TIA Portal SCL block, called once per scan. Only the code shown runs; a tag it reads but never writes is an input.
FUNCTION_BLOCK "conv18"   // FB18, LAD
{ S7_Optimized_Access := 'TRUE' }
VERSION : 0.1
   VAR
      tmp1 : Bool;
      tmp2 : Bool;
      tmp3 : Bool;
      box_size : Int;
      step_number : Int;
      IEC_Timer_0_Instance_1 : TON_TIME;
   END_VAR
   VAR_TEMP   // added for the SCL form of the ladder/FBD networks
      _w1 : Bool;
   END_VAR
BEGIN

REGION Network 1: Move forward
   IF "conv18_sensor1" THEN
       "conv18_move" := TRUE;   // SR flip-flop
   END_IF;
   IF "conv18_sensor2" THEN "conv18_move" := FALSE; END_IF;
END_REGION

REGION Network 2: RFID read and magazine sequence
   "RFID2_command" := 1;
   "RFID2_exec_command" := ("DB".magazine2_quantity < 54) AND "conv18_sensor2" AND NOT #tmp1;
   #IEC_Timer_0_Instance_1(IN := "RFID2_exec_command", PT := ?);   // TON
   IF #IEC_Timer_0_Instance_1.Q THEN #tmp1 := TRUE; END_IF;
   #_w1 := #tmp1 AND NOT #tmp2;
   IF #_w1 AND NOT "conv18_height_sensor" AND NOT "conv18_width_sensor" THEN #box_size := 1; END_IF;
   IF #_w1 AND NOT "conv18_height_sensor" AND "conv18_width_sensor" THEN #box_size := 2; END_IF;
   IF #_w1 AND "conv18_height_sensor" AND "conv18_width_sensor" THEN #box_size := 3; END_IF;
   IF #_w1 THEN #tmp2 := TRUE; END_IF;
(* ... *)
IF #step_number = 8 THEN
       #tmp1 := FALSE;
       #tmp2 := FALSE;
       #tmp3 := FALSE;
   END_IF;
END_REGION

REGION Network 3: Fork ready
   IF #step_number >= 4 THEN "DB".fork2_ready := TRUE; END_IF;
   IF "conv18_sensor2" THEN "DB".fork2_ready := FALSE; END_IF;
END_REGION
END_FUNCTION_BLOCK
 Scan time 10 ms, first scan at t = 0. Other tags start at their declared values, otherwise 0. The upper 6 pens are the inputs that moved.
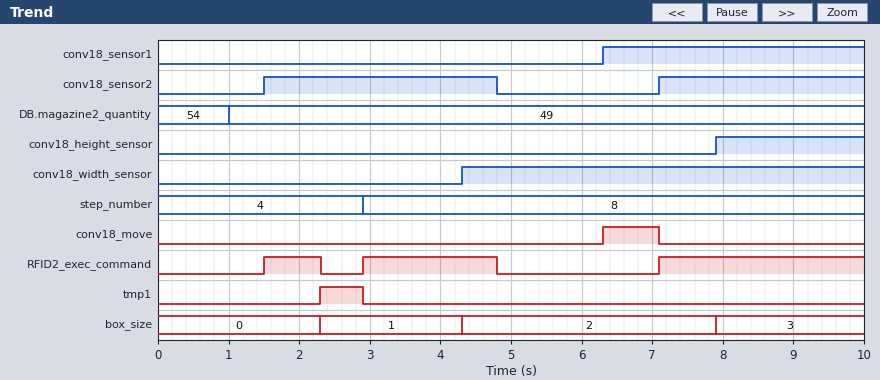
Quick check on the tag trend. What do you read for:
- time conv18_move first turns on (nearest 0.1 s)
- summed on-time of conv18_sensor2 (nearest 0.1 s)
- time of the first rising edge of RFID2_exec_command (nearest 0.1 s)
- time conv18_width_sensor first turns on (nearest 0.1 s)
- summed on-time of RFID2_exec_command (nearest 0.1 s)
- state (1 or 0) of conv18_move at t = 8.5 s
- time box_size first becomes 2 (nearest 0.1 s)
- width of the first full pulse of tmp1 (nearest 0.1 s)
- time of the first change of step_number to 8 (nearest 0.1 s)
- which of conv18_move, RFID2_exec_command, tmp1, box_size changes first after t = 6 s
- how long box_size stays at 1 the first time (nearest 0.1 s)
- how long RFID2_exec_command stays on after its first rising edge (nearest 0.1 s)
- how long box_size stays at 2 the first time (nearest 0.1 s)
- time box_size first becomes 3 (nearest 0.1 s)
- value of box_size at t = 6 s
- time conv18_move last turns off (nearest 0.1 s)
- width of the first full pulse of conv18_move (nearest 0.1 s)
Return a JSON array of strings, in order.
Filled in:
["6.3 s", "6.2 s", "1.5 s", "4.3 s", "5.6 s", "0", "4.3 s", "0.6 s", "2.9 s", "conv18_move", "2.0 s", "0.8 s", "3.6 s", "7.9 s", "2", "7.1 s", "0.8 s"]
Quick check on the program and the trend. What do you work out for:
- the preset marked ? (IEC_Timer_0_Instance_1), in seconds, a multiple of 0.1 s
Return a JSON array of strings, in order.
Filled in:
["0.8 s"]
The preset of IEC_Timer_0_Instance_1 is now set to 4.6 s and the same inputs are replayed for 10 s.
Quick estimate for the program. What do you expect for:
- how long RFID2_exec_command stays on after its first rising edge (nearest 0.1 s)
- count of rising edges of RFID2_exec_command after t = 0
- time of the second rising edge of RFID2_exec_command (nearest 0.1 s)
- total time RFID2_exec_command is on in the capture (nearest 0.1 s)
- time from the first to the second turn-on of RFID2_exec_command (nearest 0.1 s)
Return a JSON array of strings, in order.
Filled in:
["3.3 s", "2", "7.1 s", "6.2 s", "5.6 s"]
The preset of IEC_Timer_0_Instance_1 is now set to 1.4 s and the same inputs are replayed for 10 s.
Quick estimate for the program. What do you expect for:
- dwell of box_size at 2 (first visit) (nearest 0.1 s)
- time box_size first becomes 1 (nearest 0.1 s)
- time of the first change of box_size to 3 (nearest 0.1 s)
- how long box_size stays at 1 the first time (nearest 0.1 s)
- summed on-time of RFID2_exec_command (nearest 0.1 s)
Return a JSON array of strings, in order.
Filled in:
["4.2 s", "2.9 s", "8.5 s", "1.4 s", "6.2 s"]
